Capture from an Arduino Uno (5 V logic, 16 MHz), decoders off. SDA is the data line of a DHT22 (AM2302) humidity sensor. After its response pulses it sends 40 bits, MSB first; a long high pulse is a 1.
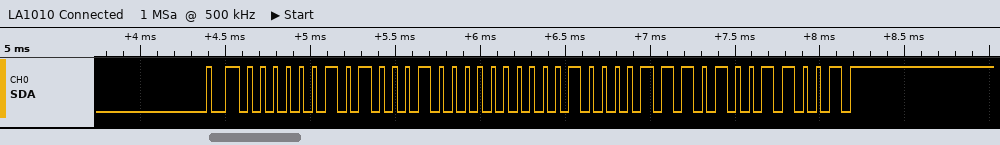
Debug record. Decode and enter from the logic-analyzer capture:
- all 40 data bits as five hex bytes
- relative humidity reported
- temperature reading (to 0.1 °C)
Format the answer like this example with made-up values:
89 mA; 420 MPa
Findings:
02 88 01 0E 99; 64.8 %; 27.0 °C
